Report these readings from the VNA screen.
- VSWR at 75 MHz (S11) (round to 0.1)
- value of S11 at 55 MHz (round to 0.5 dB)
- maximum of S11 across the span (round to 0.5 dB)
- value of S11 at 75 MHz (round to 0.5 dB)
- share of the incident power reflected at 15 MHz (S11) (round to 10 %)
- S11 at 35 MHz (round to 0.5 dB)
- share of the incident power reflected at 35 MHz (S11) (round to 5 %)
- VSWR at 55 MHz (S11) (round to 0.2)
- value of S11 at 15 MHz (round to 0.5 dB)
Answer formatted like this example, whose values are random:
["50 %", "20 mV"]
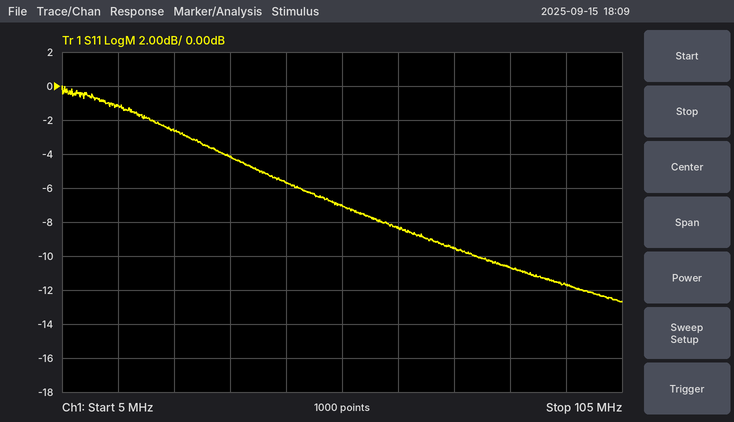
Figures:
["2.0", "-7.0 dB", "0.0 dB", "-9.5 dB", "80 %", "-4.0 dB", "40 %", "2.6", "-1.0 dB"]
